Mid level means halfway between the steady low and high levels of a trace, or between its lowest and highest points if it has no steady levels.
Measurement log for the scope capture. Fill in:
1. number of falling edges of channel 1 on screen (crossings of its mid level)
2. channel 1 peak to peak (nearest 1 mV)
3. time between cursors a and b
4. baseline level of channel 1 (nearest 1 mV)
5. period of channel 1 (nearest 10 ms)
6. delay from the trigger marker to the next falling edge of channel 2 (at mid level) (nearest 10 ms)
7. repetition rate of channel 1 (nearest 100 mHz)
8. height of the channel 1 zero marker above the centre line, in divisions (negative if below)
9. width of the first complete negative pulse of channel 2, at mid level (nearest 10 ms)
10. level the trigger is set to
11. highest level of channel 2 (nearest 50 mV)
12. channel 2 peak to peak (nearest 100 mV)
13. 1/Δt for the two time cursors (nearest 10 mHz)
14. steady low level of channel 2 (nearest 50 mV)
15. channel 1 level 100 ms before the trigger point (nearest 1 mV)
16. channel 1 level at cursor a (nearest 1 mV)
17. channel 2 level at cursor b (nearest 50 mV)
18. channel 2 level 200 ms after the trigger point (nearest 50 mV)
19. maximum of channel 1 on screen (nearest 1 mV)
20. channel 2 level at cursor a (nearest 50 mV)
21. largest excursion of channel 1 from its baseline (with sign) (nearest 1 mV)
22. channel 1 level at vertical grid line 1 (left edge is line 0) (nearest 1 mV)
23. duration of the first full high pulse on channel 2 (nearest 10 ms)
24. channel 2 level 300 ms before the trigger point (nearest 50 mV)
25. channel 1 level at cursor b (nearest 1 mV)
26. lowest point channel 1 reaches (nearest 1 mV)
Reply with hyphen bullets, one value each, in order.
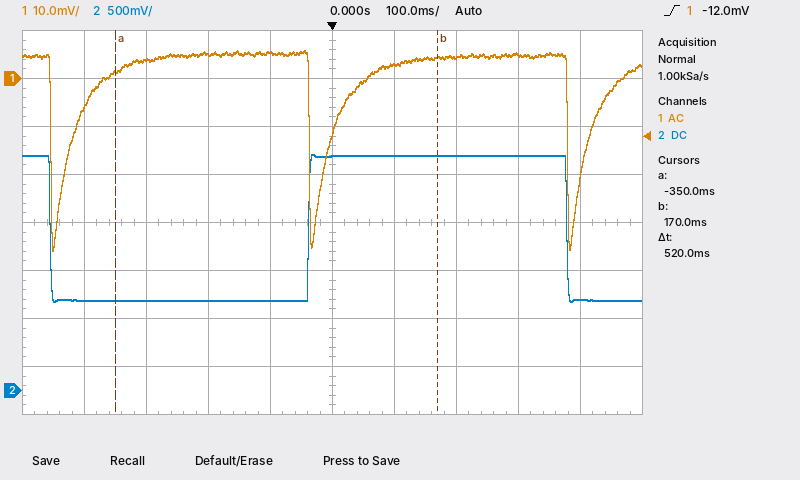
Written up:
- 3
- 42 mV
- 520 ms
- 5 mV
- 420 ms
- 380 ms
- 2.4 Hz
- +3.0 div
- 420 ms
- -12.0 mV
- 2.45 V
- 1.50 V
- 1.92 Hz
- 950 mV
- 5 mV
- 1 mV
- 2.45 V
- 2.45 V
- 6 mV
- 950 mV
- -41 mV
- -6 mV
- 420 ms
- 950 mV
- 4 mV
- -36 mV
